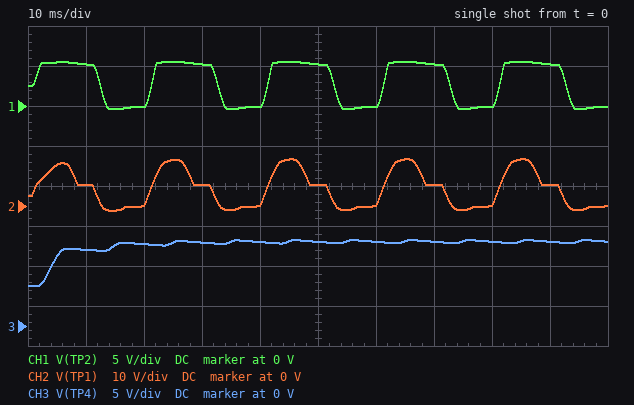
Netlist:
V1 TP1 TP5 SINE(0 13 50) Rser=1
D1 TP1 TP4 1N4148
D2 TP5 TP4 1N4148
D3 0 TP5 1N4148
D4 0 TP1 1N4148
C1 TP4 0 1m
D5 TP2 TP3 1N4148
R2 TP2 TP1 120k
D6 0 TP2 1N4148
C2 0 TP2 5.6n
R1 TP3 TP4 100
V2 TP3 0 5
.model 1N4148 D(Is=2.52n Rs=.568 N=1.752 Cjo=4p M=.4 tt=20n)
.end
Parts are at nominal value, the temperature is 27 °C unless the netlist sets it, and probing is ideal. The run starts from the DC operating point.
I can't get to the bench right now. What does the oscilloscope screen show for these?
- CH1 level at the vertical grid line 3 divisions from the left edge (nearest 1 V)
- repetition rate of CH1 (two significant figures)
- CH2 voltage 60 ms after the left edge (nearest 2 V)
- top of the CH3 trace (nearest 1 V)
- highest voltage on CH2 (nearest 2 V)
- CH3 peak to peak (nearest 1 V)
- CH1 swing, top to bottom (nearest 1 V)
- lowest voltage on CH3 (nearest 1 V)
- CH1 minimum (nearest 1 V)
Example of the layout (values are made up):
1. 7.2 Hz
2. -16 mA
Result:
1. 5 V
2. 50 Hz
3. 0 V
4. 11 V
5. 12 V
6. 6 V
7. 6 V
8. 5 V
9. 0 V
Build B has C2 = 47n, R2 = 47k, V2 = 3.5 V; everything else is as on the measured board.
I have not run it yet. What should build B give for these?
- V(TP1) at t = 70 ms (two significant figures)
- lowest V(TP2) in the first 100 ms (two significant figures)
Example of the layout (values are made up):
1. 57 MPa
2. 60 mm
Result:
1. 3.8 V
2. -320 mV
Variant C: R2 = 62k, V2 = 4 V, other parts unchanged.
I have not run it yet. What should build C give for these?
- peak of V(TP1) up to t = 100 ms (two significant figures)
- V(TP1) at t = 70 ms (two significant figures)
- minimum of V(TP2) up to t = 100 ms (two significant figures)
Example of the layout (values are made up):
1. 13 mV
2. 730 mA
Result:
1. 12 V
2. 4.2 V
3. -390 mV
